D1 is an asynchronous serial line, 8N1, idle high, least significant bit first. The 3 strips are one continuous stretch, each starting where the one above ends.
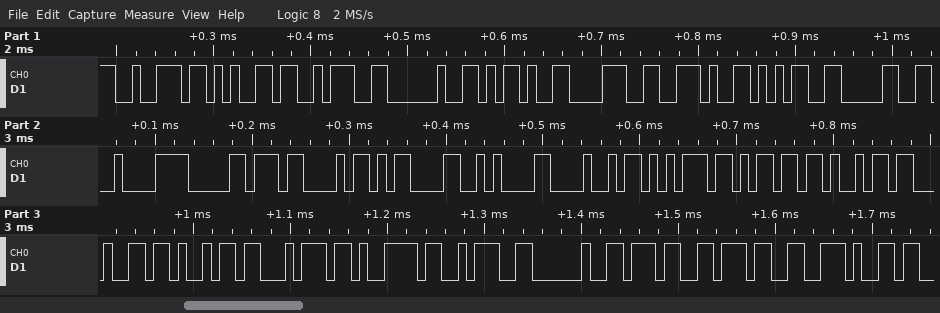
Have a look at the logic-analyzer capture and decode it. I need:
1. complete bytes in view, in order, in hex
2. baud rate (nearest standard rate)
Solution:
72 65 3A 20 2D 38 2E 35 30 C2 B0 43 0D 0A 48 75 6D 69 64 69 74 79 3A 20 37 37 2E
115200 baud
